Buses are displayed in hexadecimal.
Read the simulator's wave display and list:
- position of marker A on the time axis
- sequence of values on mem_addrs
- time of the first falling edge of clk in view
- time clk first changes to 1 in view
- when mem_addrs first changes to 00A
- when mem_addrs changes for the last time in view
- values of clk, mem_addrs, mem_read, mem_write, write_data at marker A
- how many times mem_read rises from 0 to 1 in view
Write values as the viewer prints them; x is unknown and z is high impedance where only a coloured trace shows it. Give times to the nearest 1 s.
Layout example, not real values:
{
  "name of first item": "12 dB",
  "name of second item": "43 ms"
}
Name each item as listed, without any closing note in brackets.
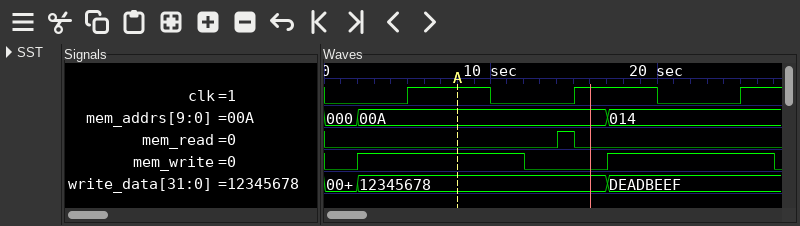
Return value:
{
  "position of marker A on the time axis": "8 s",
  "sequence of values on mem_addrs": "000, 00A, 014",
  "time of the first falling edge of clk in view": "10 s",
  "time clk first changes to 1 in view": "5 s",
  "when mem_addrs first changes to 00A": "2 s",
  "when mem_addrs changes for the last time in view": "17 s",
  "values of clk, mem_addrs, mem_read, mem_write, write_data at marker A": "clk=1, mem_addrs=00A, mem_read=0, mem_write=1, write_data=12345678",
  "how many times mem_read rises from 0 to 1 in view": "1"
}
